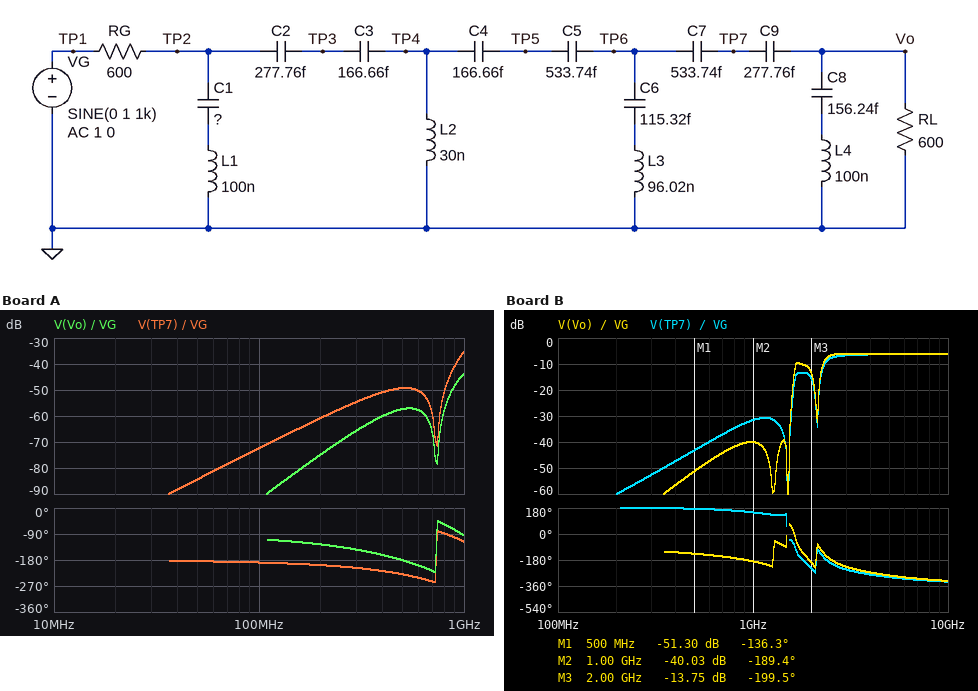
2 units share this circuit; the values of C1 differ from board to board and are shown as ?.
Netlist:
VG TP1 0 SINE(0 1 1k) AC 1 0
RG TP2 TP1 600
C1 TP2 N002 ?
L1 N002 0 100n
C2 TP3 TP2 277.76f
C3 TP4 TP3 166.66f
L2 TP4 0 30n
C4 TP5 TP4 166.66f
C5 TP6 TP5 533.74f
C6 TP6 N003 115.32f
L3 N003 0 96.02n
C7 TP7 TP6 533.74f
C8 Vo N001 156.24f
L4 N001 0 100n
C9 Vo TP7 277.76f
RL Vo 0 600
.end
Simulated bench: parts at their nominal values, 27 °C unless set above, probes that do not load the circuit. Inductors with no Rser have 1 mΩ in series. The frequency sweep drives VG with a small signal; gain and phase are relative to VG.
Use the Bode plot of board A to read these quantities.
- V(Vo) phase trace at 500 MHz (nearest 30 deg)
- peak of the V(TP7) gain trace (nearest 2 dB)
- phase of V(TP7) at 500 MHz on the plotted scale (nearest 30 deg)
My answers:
-180 deg
-36 dB
-240 deg
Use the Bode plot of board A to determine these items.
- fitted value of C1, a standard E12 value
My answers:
470 fF
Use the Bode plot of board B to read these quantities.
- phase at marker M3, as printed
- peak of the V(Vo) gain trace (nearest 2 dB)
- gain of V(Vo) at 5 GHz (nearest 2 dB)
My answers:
-199.5 deg
-6 dB
-6 dB
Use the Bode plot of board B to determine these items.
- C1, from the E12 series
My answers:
56 fF
